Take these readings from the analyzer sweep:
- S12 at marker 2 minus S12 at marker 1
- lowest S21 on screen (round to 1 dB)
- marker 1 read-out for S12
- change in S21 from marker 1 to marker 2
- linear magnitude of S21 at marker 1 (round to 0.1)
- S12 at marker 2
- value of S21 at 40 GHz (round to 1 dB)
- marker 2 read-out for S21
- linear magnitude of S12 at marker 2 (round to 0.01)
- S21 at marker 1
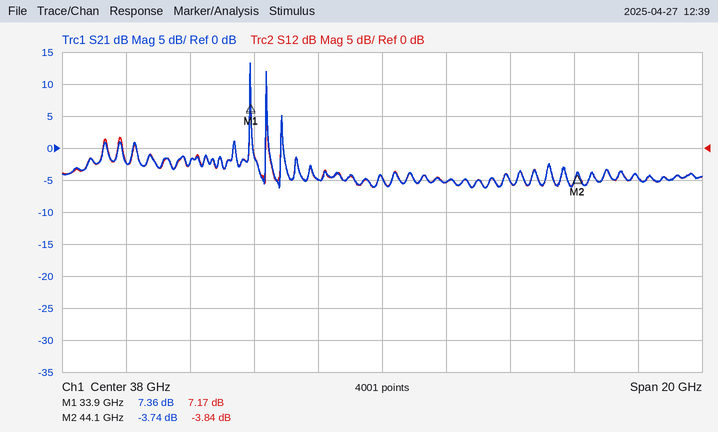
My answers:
-11.01 dB
-6 dB
7.17 dB
-11.10 dB
2.3
-3.84 dB
-5 dB
-3.74 dB
0.64
7.36 dB
